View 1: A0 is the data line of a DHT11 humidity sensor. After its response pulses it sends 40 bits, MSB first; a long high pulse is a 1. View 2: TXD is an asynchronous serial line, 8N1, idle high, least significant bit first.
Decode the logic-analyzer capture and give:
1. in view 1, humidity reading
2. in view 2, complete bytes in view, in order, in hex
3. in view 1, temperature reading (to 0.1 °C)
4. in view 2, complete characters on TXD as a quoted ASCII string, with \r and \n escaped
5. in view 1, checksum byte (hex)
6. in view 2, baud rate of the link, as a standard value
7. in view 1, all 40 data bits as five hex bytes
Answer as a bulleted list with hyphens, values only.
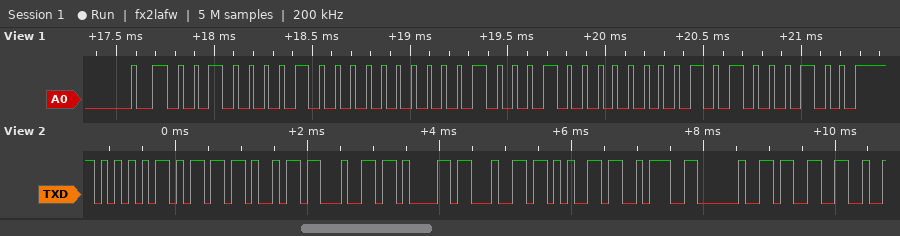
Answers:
- 33 %
- 0x55 0x6D 0x69 0x64 0x61 0x64 0x65 0x3A 0x20 0x33
- 34.1 °C
- "Umidade: 3"
- 0x44
- 9600 baud
- 21 00 22 01 44
